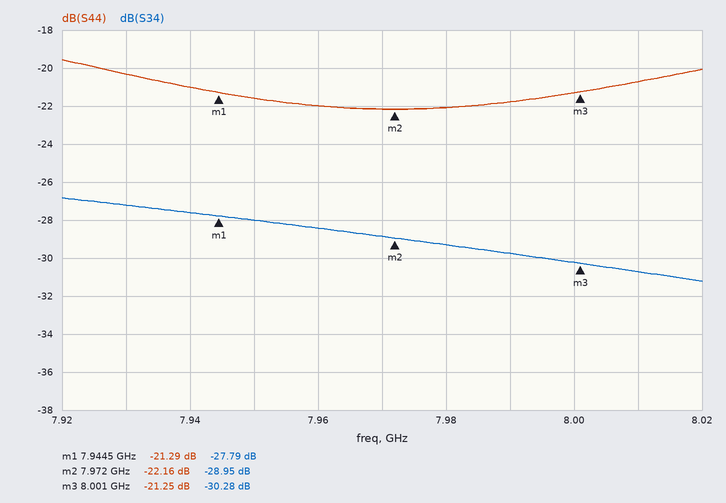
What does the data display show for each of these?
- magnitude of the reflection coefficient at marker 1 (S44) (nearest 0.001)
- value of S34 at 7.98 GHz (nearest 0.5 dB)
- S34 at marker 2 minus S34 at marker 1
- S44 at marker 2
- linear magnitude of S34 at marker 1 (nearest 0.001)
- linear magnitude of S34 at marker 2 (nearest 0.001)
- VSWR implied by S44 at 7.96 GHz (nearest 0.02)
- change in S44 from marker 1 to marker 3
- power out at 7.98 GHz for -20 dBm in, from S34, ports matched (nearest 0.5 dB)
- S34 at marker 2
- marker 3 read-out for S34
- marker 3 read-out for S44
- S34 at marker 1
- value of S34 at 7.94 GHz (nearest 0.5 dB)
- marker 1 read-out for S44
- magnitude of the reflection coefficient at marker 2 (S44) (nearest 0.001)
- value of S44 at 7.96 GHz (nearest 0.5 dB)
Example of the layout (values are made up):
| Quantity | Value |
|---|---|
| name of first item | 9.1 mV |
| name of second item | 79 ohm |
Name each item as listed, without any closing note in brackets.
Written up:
| Quantity | Value |
|---|---|
| magnitude of the reflection coefficient at marker 1 (S44) | 0.086 |
| value of S34 at 7.98 GHz | -29.5 dB |
| S34 at marker 2 minus S34 at marker 1 | -1.16 dB |
| S44 at marker 2 | -22.16 dB |
| linear magnitude of S34 at marker 1 | 0.041 |
| linear magnitude of S34 at marker 2 | 0.036 |
| VSWR implied by S44 at 7.96 GHz | 1.18 |
| change in S44 from marker 1 to marker 3 | 0.04 dB |
| power out at 7.98 GHz for -20 dBm in, from S34, ports matched | -49.5 dBm |
| S34 at marker 2 | -28.95 dB |
| marker 3 read-out for S34 | -30.28 dB |
| marker 3 read-out for S44 | -21.25 dB |
| S34 at marker 1 | -27.79 dB |
| value of S34 at 7.94 GHz | -27.5 dB |
| marker 1 read-out for S44 | -21.29 dB |
| magnitude of the reflection coefficient at marker 2 (S44) | 0.078 |
| value of S44 at 7.96 GHz | -22.0 dB |
